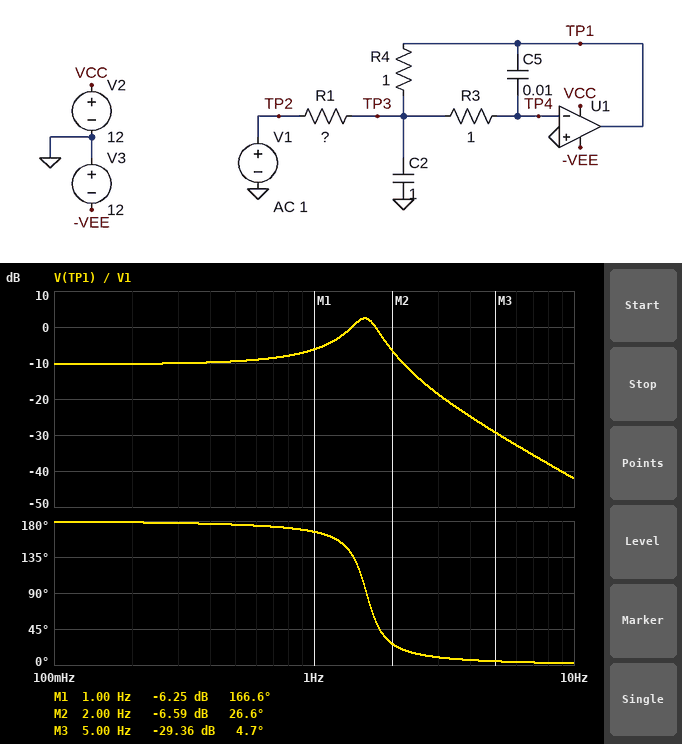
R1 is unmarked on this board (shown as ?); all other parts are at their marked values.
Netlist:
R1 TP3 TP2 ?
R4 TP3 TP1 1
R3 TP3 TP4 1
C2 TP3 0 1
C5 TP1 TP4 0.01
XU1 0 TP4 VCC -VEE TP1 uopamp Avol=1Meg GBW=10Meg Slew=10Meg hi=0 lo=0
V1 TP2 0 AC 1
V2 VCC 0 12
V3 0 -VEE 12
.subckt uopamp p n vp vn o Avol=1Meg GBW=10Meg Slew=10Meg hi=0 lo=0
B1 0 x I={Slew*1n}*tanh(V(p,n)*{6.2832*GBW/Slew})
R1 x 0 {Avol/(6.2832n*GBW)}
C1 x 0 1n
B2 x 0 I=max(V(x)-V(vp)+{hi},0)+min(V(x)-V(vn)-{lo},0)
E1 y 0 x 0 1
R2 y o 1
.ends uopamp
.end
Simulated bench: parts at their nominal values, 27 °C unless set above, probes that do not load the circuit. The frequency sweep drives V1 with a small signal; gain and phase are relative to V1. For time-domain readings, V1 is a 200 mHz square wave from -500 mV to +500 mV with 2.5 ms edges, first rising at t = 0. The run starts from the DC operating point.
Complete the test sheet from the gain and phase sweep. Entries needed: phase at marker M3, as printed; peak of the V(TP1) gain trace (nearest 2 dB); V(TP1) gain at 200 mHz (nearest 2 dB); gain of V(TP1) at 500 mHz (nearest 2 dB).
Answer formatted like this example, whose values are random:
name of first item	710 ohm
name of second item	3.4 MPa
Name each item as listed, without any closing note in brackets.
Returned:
phase at marker M3, as printed	4.7 deg
peak of the V(TP1) gain trace	2 dB
V(TP1) gain at 200 mHz	-10 dB
gain of V(TP1) at 500 mHz	-10 dB
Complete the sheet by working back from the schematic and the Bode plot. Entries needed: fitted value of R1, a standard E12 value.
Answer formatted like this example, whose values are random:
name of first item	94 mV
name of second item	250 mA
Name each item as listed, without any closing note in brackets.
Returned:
fitted value of R1, a standard E12 value	3.3 Ω
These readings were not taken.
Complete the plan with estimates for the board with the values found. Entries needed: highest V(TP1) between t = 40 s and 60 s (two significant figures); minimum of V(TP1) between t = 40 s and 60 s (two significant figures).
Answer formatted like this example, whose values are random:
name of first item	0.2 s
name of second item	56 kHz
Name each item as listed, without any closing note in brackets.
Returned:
highest V(TP1) between t = 40 s and 60 s	350 mV
minimum of V(TP1) between t = 40 s and 60 s	-350 mV
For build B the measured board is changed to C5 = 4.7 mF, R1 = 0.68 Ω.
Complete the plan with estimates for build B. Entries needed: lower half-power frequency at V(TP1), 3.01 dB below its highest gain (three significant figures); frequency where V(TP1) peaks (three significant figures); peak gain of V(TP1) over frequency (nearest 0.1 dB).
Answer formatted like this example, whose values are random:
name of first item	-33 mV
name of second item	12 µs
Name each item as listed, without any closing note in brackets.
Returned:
lower half-power frequency at V(TP1), 3.01 dB below its highest gain	1.99 Hz
frequency where V(TP1) peaks	2.29 Hz
peak gain of V(TP1) over frequency	15.9 dB
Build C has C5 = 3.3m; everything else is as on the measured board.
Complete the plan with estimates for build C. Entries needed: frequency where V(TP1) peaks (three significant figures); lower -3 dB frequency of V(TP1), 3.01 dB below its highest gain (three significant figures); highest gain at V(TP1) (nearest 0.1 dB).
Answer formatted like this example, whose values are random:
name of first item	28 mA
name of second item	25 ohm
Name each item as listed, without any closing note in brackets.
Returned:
frequency where V(TP1) peaks	2.76 Hz
lower -3 dB frequency of V(TP1), 3.01 dB below its highest gain	2.57 Hz
highest gain at V(TP1)	7.2 dB
